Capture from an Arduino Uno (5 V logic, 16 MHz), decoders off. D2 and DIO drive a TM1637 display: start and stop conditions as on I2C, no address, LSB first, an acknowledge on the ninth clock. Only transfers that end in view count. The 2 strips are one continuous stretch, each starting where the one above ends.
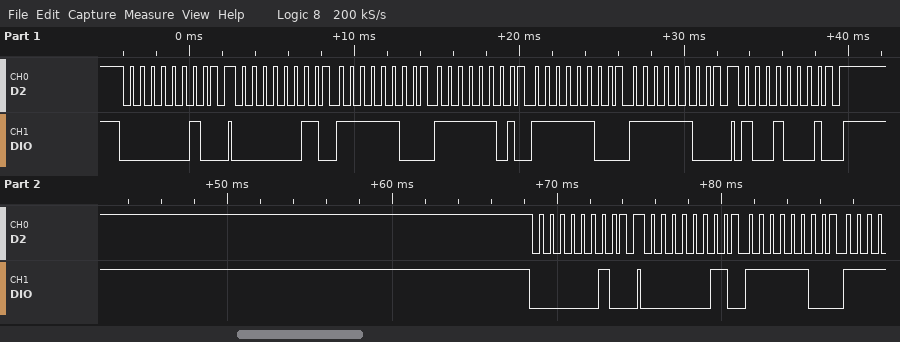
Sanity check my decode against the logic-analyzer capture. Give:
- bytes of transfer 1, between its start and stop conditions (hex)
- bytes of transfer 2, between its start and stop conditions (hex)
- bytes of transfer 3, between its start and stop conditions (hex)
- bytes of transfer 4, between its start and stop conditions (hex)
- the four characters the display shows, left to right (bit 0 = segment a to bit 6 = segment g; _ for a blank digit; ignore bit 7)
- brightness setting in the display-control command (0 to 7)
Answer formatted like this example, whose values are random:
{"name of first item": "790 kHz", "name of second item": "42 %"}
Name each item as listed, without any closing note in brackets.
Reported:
{"bytes of transfer 1, between its start and stop conditions": "40", "bytes of transfer 2, between its start and stop conditions": "C0 3F BF 3F 3F", "bytes of transfer 3, between its start and stop conditions": "89", "bytes of transfer 4, between its start and stop conditions": "40", "the four characters the display shows, left to right": "0000", "brightness setting in the display-control command": "1"}
